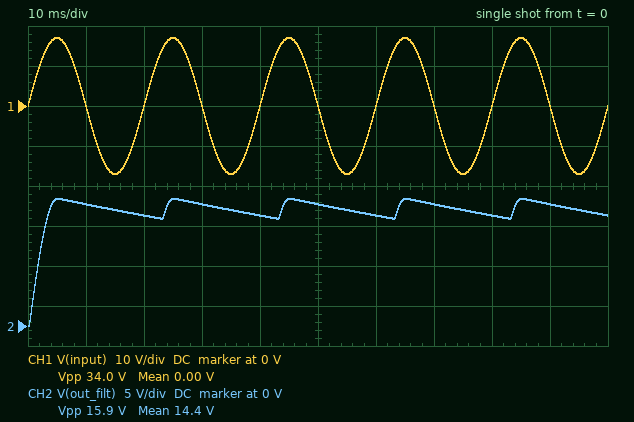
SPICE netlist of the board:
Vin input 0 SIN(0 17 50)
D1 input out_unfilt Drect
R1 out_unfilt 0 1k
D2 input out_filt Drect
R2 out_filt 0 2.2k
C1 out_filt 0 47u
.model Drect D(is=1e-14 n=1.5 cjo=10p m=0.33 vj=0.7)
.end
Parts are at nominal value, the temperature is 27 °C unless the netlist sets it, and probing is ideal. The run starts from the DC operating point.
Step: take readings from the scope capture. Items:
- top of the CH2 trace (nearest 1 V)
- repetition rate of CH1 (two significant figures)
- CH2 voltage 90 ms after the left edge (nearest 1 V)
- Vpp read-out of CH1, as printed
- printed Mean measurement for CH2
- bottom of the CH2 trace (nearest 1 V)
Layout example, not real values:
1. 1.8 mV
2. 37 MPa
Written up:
1. 16 V
2. 50 Hz
3. 15 V
4. 34.0 V
5. 14.4 V
6. 0 V
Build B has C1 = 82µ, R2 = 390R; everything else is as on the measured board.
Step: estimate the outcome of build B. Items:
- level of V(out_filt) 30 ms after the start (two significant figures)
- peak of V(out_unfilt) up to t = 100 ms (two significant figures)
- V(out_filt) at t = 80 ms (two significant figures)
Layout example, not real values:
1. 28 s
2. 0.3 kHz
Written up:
1. 14 V
2. 16 V
3. 10 V
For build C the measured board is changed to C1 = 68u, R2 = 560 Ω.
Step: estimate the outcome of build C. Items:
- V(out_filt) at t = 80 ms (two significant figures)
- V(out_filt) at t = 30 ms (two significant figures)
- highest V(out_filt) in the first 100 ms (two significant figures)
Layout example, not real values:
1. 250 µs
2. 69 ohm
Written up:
1. 11 V
2. 14 V
3. 16 V
